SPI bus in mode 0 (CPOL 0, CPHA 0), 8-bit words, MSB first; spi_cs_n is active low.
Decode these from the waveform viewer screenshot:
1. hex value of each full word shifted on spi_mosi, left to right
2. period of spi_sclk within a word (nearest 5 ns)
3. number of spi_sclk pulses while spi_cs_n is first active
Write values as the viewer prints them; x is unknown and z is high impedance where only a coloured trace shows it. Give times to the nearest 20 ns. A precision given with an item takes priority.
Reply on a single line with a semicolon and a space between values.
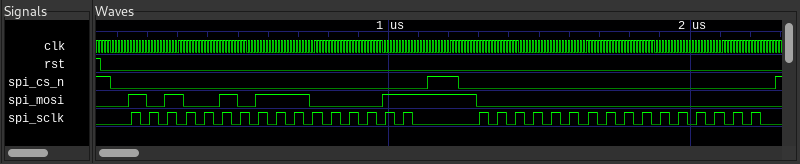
A5, C3, 00, 00; 60 ns; 16
